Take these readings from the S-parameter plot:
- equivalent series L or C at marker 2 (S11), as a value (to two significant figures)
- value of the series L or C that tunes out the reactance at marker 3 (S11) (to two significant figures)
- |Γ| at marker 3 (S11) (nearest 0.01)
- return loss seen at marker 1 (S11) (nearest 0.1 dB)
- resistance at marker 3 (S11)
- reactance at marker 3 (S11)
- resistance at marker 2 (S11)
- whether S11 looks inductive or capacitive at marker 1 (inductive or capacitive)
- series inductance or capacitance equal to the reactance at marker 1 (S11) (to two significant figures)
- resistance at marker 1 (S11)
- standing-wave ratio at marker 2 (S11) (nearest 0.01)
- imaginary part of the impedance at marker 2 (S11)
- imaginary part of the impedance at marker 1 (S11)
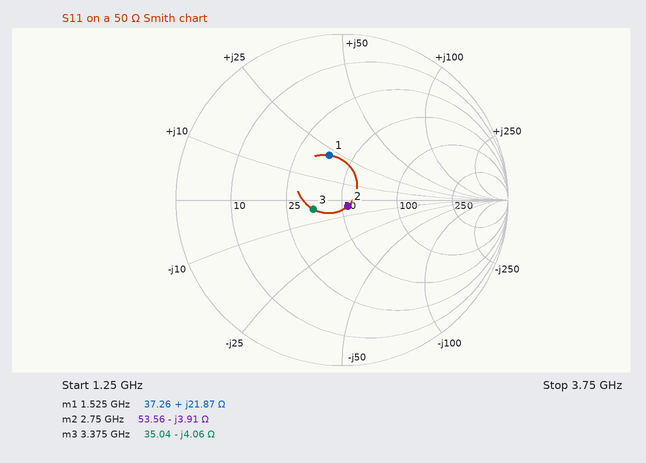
15 pF
190 pH
0.18
11.0 dB
35.04 Ω
-4.06 Ω
53.56 Ω
inductive
2.3 nH
37.26 Ω
1.11
-3.91 Ω
+21.87 Ω
